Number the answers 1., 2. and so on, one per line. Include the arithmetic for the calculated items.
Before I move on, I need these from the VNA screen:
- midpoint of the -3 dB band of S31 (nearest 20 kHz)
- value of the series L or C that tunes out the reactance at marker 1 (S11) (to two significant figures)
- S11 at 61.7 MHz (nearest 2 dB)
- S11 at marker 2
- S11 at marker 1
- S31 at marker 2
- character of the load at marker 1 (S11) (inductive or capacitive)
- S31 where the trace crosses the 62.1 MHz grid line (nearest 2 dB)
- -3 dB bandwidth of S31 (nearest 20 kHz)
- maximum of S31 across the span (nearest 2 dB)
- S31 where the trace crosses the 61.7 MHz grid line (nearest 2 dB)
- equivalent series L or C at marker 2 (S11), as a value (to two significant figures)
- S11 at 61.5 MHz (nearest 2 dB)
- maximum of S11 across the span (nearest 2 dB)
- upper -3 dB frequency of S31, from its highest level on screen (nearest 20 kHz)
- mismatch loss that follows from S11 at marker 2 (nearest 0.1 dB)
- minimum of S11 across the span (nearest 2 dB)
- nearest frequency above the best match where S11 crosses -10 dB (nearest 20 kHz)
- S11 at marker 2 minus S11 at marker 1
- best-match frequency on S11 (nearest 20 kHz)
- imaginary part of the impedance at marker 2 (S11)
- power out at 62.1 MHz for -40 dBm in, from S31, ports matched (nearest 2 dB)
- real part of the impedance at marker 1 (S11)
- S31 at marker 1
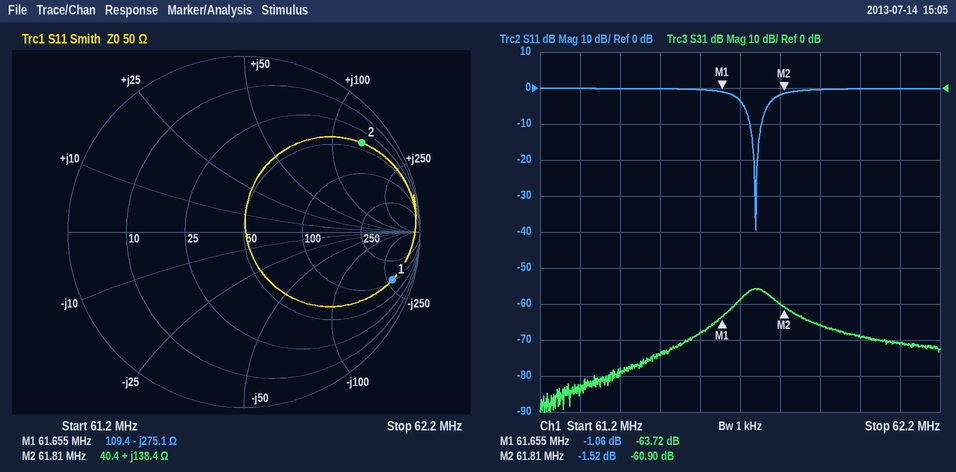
1. 61.74 MHz
2. L = 275.1 Ω/(2π × 61.655 MHz) ≈ 710 nH
3. -4 dB
4. -1.52 dB
5. -1.06 dB
6. -60.90 dB
7. capacitive
8. -70 dB
9. 61.78 MHz − 61.70 MHz = 80 kHz
10. -56 dB
11. -58 dB
12. L = 138.4 Ω/(2π × 61.81 MHz) ≈ 356 nH, so 360 nH to two significant figures
13. 0 dB
14. 0 dB
15. 61.78 MHz
16. −10 log10(1 − 10^(-1.52/10)) ≈ 5.3 dB
17. -40 dB
18. 61.76 MHz
19. -1.52 − (-1.06) = -0.46 dB
20. 61.74 MHz
21. +138.4 Ω
22. -40 dBm + (-70 dB) = -110 dBm
23. 109.4 Ω
24. -63.72 dB
